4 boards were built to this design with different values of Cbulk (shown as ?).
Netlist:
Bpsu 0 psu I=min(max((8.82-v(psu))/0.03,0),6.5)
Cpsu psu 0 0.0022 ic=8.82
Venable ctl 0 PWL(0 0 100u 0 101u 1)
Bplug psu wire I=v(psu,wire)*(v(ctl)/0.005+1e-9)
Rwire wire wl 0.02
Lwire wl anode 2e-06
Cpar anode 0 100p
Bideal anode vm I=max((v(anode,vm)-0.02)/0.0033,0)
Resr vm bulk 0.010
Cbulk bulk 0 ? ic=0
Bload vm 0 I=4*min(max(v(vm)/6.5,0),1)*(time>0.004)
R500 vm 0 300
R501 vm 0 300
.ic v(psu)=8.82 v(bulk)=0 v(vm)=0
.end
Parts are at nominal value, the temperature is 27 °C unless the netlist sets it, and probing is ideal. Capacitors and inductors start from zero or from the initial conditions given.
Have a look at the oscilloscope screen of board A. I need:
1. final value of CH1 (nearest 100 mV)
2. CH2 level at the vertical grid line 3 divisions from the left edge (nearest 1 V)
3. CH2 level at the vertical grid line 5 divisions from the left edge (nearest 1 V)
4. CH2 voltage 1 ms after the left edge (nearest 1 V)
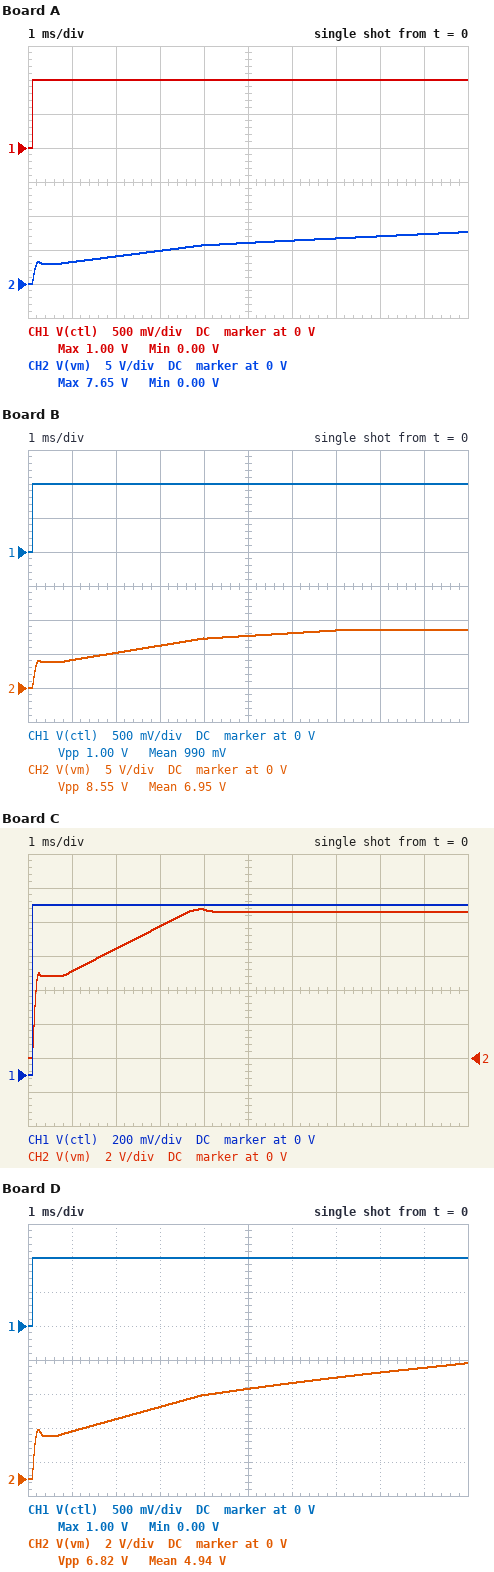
1.0 V
5 V
6 V
3 V
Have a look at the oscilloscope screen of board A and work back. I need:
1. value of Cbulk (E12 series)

5.6 mF
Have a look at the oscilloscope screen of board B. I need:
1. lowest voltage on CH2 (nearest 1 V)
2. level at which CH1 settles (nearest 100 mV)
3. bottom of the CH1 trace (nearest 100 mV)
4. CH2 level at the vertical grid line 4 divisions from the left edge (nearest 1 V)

0 V
1.0 V
0 V
7 V
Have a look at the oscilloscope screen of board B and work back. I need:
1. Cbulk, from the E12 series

3.9 mF
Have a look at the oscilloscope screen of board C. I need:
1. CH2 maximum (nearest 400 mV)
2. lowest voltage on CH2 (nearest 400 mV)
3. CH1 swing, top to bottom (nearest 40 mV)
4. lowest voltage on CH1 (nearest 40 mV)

8.8 V
0 V
1.00 V
0 V
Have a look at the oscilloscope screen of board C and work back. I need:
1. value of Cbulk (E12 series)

2.7 mF
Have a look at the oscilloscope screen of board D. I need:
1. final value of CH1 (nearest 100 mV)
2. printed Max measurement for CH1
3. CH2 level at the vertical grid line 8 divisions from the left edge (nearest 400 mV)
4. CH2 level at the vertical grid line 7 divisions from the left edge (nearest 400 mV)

1.0 V
1.00 V
6.4 V
6.0 V
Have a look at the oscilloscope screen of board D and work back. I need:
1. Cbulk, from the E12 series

6.8 mF
